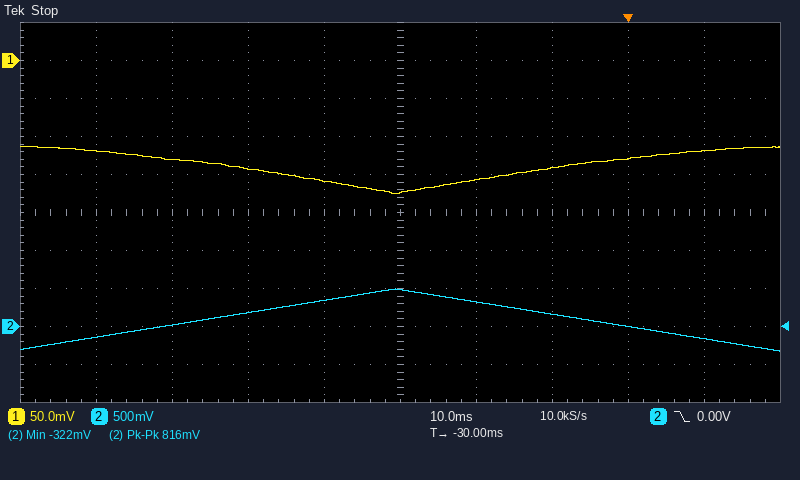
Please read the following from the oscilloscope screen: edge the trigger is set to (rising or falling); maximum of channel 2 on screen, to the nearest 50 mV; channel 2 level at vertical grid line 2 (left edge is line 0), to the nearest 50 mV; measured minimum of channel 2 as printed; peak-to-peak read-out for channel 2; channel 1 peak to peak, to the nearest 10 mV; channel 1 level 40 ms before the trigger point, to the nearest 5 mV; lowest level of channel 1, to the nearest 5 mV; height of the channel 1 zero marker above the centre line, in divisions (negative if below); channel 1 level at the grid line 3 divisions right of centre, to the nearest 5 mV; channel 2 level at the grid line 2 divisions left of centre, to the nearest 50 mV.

falling
500 mV
0 mV
-322 mV
816 mV
60 mV
-160 mV
-175 mV
+4.0 div
-130 mV
200 mV
